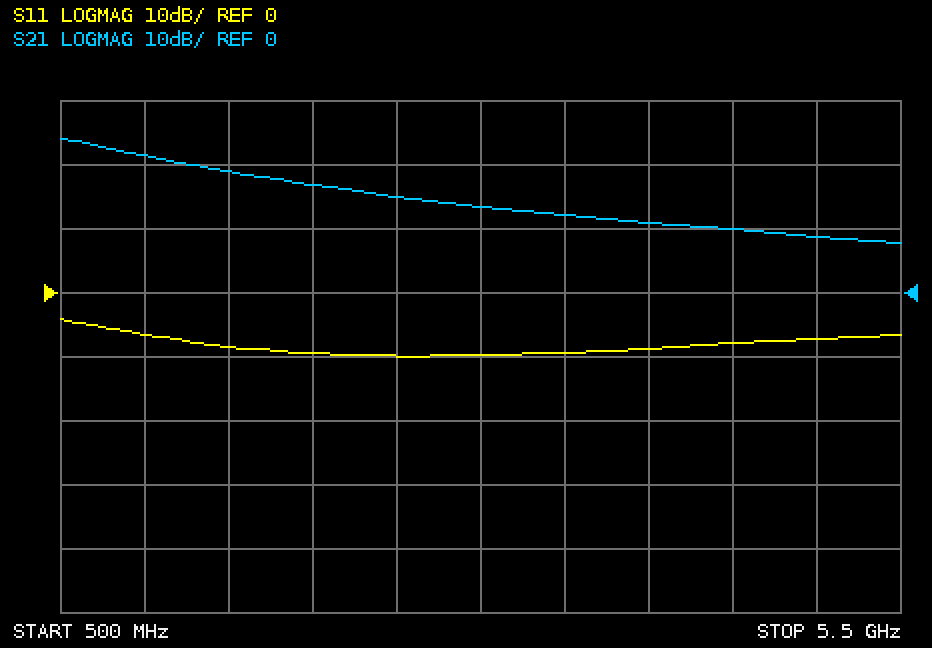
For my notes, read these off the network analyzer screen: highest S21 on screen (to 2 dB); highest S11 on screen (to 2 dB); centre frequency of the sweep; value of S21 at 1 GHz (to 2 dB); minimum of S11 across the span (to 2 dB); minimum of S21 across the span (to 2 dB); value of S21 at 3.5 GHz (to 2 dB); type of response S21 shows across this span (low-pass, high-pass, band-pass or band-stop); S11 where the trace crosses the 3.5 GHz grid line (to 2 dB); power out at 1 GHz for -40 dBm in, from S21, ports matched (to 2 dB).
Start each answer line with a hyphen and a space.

- 24 dB
- -4 dB
- 3 GHz
- 22 dB
- -10 dB
- 8 dB
- 12 dB
- low-pass
- -10 dB
- -18 dBm
